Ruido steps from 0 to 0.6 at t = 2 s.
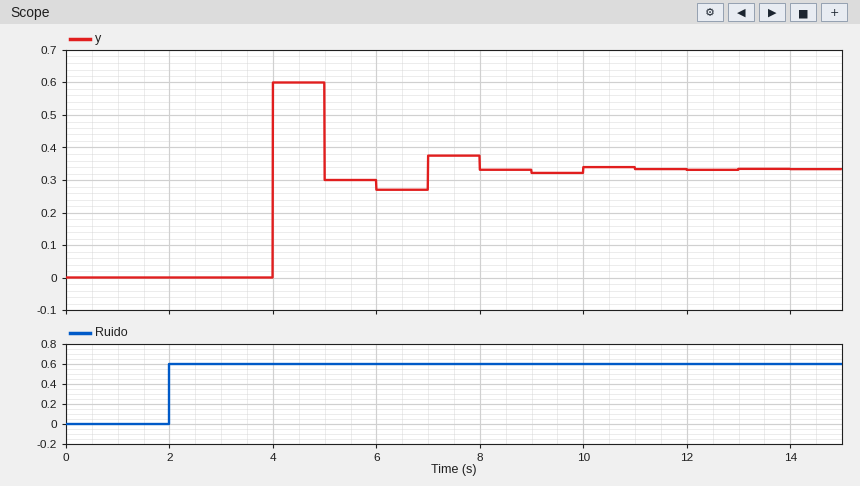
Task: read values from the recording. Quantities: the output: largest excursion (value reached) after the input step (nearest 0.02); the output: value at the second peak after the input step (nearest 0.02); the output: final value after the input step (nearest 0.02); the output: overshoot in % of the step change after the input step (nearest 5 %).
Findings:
0.60
0.38
0.34
80 %
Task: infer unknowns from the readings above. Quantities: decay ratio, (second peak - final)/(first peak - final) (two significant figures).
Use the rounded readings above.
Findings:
0.15
